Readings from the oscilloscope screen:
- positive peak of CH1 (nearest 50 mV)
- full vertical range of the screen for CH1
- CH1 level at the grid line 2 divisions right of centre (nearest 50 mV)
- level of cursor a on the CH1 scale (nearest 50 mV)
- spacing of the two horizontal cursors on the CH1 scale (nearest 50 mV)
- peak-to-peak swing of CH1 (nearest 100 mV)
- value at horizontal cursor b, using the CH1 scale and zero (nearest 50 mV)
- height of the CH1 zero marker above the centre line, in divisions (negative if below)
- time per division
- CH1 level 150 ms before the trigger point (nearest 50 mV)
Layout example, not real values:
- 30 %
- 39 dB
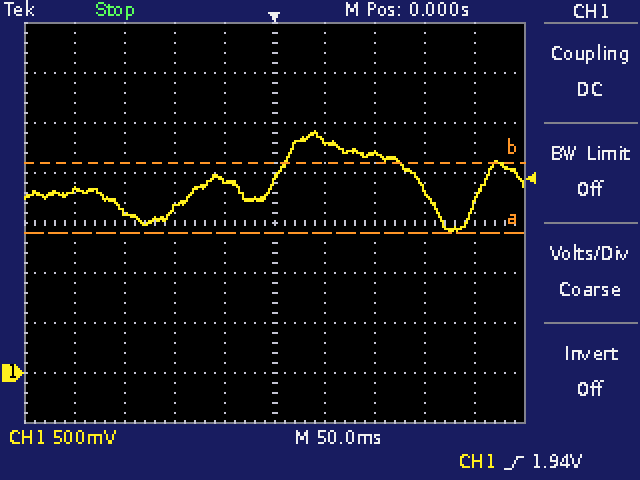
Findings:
- 2.40 V
- 4 V
- 2.20 V
- 1.40 V
- 700 mV
- 1.00 V
- 2.10 V
- -3.0 div
- 50 ms
- 1.60 V
